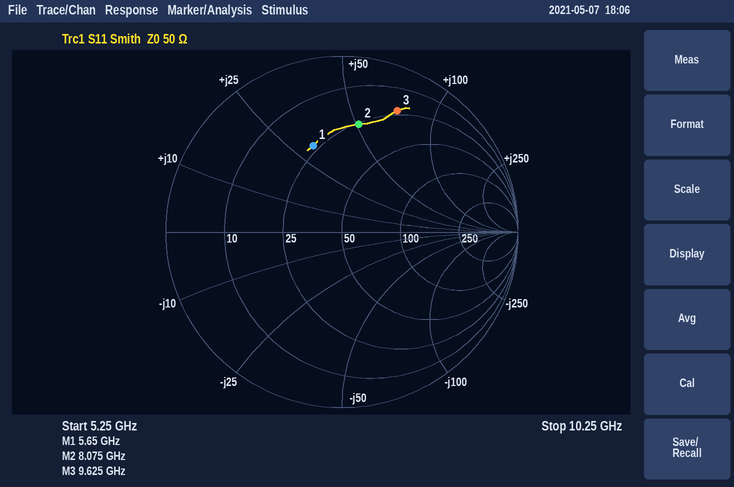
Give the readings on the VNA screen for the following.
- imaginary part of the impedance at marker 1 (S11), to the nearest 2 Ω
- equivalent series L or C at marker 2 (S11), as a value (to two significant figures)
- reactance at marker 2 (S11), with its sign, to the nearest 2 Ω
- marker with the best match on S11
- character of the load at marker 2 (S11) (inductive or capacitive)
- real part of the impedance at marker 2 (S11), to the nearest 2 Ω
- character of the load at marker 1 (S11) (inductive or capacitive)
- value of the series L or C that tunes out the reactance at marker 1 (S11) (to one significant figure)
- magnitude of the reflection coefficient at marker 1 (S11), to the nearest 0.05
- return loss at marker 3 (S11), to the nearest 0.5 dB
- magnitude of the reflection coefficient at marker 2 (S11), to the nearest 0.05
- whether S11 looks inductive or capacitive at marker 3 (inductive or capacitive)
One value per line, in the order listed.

+30 Ω
1.0 nH
+52 Ω
marker 1
inductive
26 Ω
inductive
900 fF
0.50
2.5 dB
0.60
inductive
